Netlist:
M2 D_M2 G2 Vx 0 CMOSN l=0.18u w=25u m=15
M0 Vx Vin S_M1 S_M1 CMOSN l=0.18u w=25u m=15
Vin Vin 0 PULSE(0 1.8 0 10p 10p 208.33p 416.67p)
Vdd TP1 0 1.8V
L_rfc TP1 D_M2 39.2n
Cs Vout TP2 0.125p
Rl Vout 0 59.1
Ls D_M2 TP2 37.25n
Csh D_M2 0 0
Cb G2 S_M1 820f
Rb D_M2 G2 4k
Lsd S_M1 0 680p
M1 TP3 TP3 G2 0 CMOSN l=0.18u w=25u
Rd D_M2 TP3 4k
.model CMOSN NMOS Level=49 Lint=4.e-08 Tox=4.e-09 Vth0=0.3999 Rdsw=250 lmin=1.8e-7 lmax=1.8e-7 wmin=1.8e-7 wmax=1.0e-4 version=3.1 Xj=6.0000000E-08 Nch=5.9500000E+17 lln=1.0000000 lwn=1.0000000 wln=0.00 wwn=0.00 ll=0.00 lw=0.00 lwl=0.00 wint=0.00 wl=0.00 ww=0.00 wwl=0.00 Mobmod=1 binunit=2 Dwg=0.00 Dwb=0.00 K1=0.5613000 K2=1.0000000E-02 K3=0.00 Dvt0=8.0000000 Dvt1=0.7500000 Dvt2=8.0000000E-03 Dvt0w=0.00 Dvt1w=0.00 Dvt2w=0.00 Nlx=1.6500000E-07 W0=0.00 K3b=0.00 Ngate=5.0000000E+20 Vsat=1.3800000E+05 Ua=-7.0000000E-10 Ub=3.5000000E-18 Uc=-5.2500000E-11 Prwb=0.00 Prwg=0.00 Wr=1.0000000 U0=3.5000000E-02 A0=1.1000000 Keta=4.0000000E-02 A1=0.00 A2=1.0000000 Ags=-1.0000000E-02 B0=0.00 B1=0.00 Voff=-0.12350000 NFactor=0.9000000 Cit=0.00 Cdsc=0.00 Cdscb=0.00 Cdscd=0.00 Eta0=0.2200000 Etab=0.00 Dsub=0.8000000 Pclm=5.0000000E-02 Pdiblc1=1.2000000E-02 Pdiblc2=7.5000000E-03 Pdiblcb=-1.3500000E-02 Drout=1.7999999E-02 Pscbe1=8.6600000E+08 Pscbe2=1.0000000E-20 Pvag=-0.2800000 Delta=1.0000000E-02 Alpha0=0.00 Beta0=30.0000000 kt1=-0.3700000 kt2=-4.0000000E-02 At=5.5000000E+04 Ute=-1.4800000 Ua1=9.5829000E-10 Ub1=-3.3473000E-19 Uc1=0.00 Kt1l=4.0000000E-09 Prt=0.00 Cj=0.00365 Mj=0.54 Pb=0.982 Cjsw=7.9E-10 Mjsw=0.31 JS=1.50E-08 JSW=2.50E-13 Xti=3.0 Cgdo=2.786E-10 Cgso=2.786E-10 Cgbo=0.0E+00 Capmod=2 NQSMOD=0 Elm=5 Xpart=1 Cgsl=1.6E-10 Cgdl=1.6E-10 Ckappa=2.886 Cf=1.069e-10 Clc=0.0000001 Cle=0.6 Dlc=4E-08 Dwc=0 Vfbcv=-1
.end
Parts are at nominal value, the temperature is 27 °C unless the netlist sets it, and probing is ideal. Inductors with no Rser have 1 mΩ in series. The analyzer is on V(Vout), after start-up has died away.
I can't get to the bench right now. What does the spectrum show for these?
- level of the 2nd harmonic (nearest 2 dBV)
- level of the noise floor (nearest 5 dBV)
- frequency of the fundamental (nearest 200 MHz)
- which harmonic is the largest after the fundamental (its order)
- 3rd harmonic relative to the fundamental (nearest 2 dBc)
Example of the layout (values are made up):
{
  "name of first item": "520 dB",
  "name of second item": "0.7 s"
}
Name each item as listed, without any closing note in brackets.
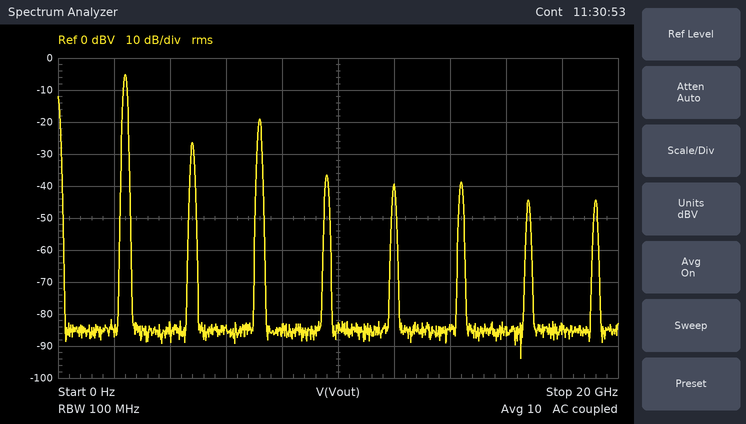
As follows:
{
  "level of the 2nd harmonic": "-26 dBV",
  "level of the noise floor": "-85 dBV",
  "frequency of the fundamental": "2.4 GHz",
  "which harmonic is the largest after the fundamental": "3",
  "3rd harmonic relative to the fundamental": "-14 dBc"
}
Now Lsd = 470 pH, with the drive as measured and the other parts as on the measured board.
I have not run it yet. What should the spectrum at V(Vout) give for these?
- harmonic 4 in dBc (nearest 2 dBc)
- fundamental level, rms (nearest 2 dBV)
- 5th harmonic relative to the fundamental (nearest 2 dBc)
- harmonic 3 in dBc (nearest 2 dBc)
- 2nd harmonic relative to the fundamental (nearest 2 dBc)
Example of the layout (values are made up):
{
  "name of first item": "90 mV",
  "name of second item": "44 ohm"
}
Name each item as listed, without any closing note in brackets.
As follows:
{
  "harmonic 4 in dBc": "-34 dBc",
  "fundamental level, rms": "0 dBV",
  "5th harmonic relative to the fundamental": "-38 dBc",
  "harmonic 3 in dBc": "-20 dBc",
  "2nd harmonic relative to the fundamental": "-26 dBc"
}
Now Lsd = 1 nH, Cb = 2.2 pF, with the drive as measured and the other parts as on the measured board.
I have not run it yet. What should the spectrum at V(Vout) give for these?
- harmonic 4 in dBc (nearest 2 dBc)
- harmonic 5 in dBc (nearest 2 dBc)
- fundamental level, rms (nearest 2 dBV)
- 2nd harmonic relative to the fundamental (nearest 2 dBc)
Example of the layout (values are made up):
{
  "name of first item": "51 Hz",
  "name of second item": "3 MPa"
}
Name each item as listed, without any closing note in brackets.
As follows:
{
  "harmonic 4 in dBc": "-38 dBc",
  "harmonic 5 in dBc": "-42 dBc",
  "fundamental level, rms": "4 dBV",
  "2nd harmonic relative to the fundamental": "-24 dBc"
}
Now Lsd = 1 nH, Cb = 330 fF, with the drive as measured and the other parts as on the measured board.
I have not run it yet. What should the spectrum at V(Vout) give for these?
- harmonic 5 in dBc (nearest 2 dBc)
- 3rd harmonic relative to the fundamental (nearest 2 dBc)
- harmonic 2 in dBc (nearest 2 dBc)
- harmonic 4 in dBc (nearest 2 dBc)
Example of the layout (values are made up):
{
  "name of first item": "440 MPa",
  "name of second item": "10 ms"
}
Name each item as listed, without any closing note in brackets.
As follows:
{
  "harmonic 5 in dBc": "-44 dBc",
  "3rd harmonic relative to the fundamental": "-30 dBc",
  "harmonic 2 in dBc": "-22 dBc",
  "harmonic 4 in dBc": "-44 dBc"
}
